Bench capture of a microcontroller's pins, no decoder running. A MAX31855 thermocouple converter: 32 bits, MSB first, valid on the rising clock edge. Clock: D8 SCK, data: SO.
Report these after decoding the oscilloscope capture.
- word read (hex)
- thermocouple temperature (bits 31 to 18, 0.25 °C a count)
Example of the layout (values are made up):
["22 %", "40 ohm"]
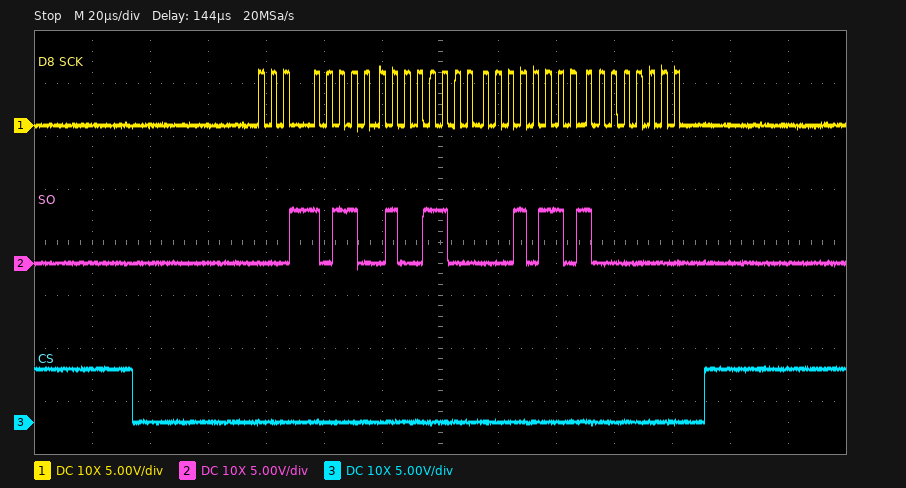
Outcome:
["0x164C1680", "356.75 °C"]
